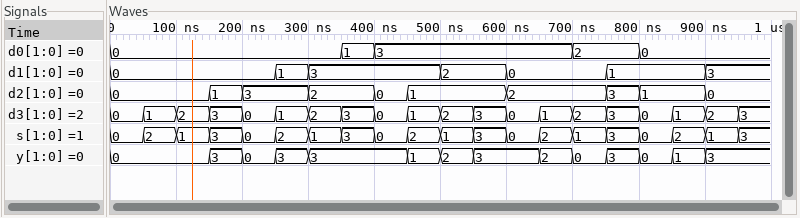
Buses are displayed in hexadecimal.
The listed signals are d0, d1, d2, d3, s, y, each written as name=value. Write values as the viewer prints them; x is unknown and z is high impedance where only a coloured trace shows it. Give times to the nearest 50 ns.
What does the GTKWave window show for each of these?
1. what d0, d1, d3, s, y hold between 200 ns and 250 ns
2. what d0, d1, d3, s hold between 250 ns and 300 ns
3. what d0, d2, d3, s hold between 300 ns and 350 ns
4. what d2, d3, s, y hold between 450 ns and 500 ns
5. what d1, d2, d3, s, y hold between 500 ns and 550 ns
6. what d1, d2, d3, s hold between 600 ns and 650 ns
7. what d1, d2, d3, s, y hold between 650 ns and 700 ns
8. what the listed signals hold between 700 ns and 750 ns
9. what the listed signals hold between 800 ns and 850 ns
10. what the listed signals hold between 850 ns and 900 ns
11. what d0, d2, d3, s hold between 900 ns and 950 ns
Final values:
d0=0, d1=0, d3=0, s=0, y=0
d0=0, d1=1, d3=1, s=2
d0=0, d2=2, d3=2, s=1
d2=1, d3=1, s=2, y=1
d1=2, d2=1, d3=2, s=1, y=2
d1=0, d2=2, d3=0, s=0
d1=0, d2=2, d3=1, s=2, y=2
d0=2, d1=0, d2=2, d3=2, s=1, y=0
d0=0, d1=1, d2=1, d3=0, s=0, y=0
d0=0, d1=1, d2=1, d3=1, s=2, y=1
d0=0, d2=0, d3=2, s=1
